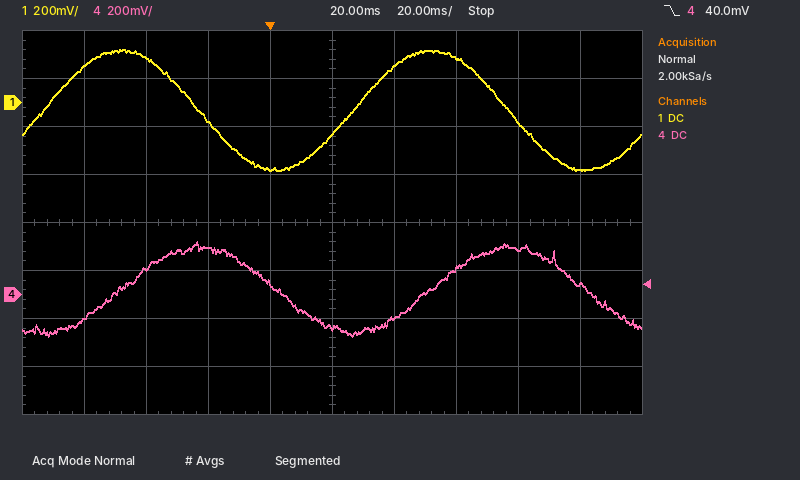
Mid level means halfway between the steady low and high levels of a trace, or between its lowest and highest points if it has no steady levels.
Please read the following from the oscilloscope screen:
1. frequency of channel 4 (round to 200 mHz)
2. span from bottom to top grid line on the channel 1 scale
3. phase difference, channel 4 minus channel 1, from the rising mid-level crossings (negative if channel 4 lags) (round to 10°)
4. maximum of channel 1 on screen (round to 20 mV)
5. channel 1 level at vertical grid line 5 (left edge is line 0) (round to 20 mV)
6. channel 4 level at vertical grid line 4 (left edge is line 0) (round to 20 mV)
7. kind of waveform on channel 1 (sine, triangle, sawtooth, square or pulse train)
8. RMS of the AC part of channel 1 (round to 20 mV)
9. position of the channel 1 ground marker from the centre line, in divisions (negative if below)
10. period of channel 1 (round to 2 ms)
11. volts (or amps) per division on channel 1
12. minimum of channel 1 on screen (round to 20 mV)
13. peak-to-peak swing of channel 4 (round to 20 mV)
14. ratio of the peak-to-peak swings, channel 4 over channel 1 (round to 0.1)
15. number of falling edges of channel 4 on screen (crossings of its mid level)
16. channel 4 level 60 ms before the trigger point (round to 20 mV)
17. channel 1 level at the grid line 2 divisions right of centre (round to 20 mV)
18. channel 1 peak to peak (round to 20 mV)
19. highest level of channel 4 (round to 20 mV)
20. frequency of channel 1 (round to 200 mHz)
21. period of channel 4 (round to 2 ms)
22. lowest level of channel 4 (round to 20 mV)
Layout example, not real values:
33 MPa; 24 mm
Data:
10.0 Hz; 1.6 V; -90°; 220 mV; -140 mV; 40 mV; sine; 180 mV; +2.5 div; 100 ms; 200 mV; -280 mV; 400 mV; 0.8; 2; -100 mV; 180 mV; 500 mV; 220 mV; 10.0 Hz; 100 ms; -180 mV
